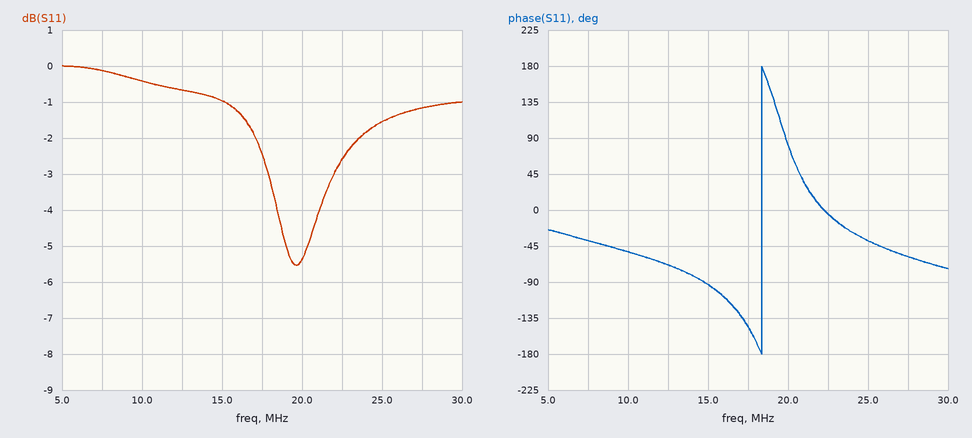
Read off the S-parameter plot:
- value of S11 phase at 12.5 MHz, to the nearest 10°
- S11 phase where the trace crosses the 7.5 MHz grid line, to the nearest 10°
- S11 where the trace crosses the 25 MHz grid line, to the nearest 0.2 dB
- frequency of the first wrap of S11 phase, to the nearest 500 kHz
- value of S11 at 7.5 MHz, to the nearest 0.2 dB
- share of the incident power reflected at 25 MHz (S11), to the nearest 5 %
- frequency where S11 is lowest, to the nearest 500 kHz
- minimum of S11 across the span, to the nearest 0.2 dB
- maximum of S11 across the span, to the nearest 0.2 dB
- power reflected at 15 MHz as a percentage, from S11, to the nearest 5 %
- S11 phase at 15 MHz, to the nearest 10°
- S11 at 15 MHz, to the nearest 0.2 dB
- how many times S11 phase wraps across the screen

-70°
-40°
-1.6 dB
18.5 MHz
-0.2 dB
70 %
19.5 MHz
-5.6 dB
0.0 dB
80 %
-90°
-1.0 dB
1
